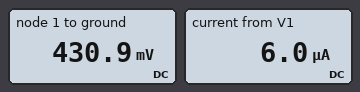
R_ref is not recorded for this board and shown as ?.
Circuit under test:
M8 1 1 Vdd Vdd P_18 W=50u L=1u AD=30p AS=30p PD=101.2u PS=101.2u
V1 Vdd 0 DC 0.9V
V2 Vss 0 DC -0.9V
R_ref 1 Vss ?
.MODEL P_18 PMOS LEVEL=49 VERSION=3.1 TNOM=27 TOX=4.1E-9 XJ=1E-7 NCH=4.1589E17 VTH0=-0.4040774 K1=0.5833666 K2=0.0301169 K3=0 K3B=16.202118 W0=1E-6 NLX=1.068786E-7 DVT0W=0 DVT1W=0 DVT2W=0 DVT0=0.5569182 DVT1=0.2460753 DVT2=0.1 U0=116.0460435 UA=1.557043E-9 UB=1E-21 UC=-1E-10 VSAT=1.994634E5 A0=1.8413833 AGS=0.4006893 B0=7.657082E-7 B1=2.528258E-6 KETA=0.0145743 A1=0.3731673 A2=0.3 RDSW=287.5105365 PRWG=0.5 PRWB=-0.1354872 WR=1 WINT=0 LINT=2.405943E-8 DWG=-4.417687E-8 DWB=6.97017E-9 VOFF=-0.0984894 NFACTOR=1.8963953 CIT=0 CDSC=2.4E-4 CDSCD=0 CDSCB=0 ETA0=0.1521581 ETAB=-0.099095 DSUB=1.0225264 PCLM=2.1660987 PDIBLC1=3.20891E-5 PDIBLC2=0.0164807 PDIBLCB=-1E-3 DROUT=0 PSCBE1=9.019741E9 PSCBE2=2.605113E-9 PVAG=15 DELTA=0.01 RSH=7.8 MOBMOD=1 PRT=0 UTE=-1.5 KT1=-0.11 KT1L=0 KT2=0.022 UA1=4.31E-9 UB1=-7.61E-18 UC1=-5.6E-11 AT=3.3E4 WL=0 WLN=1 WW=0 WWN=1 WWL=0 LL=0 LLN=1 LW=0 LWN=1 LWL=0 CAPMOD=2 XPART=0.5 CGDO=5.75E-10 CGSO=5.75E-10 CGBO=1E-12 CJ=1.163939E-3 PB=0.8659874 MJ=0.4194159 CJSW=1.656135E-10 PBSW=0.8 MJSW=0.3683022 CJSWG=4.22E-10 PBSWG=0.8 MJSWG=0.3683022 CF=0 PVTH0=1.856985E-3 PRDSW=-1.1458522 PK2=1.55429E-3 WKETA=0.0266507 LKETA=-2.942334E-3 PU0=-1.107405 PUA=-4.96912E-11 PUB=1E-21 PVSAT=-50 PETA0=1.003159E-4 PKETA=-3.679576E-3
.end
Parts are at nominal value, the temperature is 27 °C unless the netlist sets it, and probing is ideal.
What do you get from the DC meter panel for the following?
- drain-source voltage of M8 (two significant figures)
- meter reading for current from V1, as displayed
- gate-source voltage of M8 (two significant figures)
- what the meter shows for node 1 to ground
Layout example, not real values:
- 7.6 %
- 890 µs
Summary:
- -470 mV
- 6.0 µA
- -470 mV
- 430.9 mV
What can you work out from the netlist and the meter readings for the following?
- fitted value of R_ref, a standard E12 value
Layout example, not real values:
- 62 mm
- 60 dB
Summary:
- 220 kΩ
